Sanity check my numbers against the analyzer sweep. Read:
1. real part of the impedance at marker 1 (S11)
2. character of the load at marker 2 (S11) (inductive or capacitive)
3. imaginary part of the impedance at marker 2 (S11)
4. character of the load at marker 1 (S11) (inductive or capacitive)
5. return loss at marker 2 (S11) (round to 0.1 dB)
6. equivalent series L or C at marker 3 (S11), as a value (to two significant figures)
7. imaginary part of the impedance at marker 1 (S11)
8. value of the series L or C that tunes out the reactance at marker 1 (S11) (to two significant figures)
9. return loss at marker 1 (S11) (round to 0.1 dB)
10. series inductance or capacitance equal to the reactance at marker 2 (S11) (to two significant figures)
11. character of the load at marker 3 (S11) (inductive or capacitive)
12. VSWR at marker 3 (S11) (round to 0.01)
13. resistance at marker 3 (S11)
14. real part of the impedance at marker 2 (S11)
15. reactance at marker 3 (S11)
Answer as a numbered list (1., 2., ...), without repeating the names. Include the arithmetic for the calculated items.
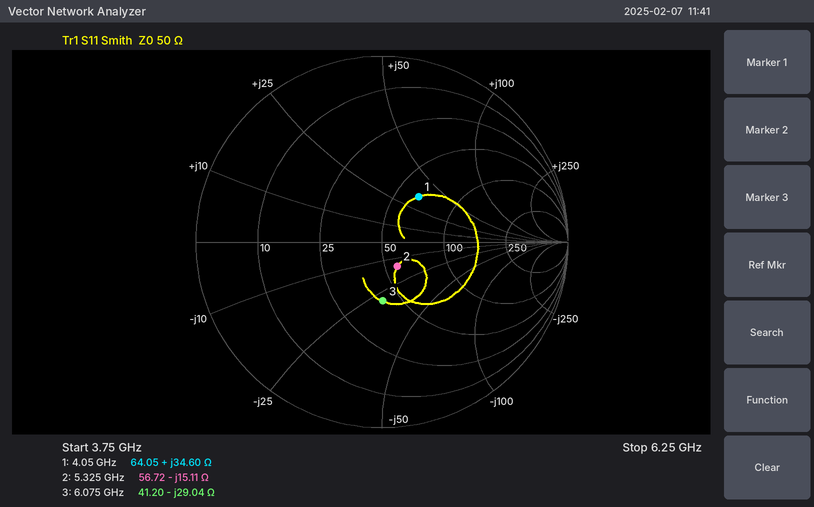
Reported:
1. 64.05 Ω
2. capacitive
3. -15.11 Ω
4. inductive
5. 16.3 dB
6. C = 1/(2π × 6.075 GHz × 29.04 Ω) ≈ 902 fF, so 900 fF to two significant figures
7. +34.60 Ω
8. C = 1/(2π × 4.05 GHz × 34.6 Ω) ≈ 1.1 pF
9. 10.1 dB
10. C = 1/(2π × 5.325 GHz × 15.11 Ω) ≈ 2.0 pF
11. capacitive
12. 1.93
13. 41.20 Ω
14. 56.72 Ω
15. -29.04 Ω
